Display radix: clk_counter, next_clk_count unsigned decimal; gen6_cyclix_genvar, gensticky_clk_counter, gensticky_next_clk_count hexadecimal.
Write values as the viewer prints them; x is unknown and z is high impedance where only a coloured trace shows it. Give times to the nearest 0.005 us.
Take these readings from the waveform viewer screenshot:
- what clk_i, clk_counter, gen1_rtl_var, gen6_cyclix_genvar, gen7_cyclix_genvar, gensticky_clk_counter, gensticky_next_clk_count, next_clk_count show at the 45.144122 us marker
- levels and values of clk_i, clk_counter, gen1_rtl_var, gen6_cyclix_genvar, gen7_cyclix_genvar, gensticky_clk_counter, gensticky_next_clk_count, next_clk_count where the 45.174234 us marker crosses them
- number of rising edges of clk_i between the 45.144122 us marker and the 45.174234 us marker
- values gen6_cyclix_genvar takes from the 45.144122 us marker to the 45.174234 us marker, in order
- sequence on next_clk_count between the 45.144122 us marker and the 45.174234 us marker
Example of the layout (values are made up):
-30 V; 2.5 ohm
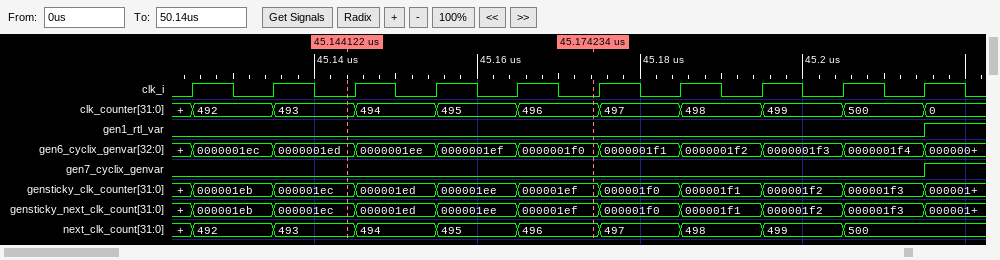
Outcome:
clk_i=0, clk_counter=493, gen1_rtl_var=0, gen6_cyclix_genvar=0000001ed, gen7_cyclix_genvar=0, gensticky_clk_counter=000001ec, gensticky_next_clk_count=000001ec, next_clk_count=493; clk_i=0, clk_counter=496, gen1_rtl_var=0, gen6_cyclix_genvar=0000001f0, gen7_cyclix_genvar=0, gensticky_clk_counter=000001ef, gensticky_next_clk_count=000001ef, next_clk_count=496; 3; 0000001ed, 0000001ee, 0000001ef, 0000001f0; 493, 494, 495, 496
